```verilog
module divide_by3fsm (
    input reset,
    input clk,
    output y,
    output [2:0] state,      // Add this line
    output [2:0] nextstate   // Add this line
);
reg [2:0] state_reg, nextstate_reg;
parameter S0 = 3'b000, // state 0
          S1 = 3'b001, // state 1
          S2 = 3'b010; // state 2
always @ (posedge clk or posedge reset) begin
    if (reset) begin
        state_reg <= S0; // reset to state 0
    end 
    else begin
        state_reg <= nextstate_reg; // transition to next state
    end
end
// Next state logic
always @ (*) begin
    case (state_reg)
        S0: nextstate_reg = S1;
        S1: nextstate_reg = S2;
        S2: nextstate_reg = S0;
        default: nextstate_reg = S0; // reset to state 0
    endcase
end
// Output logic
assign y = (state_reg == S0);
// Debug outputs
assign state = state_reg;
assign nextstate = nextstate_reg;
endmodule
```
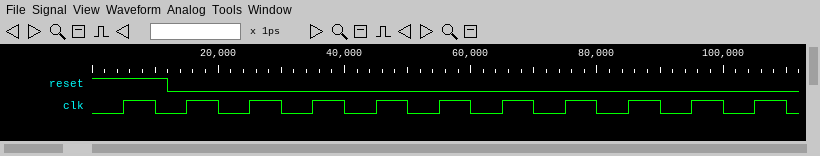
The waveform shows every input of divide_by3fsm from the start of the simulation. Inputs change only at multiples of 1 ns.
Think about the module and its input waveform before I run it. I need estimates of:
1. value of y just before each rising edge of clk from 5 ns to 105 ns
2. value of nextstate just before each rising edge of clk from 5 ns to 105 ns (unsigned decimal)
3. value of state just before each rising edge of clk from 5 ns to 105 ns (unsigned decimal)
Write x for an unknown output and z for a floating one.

1 1 0 0 1 0 0 1 0 0 1
1, 1, 2, 0, 1, 2, 0, 1, 2, 0, 1
0, 0, 1, 2, 0, 1, 2, 0, 1, 2, 0
